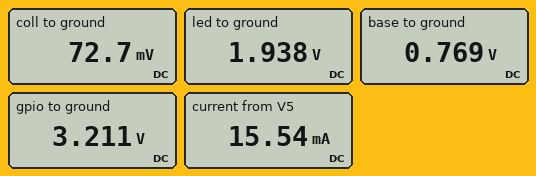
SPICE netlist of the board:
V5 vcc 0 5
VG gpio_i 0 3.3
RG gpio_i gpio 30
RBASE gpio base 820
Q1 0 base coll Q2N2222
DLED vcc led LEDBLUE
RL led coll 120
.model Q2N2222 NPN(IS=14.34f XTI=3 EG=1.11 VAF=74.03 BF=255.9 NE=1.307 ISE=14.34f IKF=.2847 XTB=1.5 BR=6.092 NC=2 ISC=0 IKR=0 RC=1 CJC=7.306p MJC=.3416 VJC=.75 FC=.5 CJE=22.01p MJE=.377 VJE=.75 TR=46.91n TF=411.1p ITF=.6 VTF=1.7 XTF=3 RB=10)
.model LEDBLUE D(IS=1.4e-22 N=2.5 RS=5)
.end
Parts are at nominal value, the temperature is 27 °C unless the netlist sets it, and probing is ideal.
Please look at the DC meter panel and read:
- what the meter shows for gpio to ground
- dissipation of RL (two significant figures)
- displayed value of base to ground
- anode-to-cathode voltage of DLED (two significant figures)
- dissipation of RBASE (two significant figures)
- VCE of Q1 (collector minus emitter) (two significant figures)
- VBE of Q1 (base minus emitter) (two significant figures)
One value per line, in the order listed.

3.211 V
29 mW
0.769 V
3.1 V
7.3 mW
-73 mV
700 mV
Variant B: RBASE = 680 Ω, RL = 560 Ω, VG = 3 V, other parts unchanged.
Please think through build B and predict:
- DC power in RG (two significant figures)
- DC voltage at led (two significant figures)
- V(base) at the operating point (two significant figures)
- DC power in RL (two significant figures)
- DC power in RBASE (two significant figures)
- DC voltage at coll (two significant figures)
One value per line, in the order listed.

300 µW
2.1 V
760 mV
7.7 mW
6.8 mW
13 mV
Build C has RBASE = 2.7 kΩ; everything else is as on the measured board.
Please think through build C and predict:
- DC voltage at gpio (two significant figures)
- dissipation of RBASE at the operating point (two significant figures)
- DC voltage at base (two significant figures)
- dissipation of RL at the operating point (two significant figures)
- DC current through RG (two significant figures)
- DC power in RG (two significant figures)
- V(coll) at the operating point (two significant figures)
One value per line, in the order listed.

3.3 V
2.4 mW
710 mV
3.9 mW
950 µA
27 µW
1.4 V
